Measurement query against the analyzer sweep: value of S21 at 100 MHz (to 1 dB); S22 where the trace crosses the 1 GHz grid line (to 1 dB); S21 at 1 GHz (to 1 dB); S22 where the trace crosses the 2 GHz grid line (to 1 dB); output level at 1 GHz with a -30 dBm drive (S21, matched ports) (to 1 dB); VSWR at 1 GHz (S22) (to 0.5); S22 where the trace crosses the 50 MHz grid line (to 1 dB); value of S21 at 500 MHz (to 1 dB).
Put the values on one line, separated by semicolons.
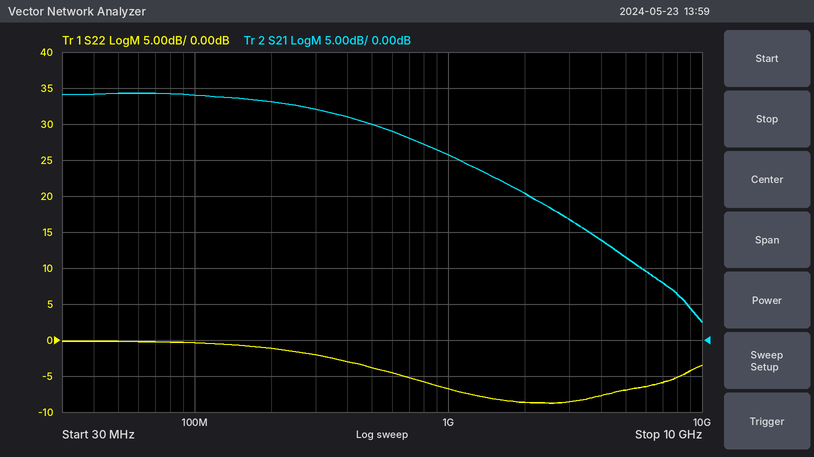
34 dB; -7 dB; 26 dB; -9 dB; -4 dBm; 2.5; 0 dB; 30 dB
